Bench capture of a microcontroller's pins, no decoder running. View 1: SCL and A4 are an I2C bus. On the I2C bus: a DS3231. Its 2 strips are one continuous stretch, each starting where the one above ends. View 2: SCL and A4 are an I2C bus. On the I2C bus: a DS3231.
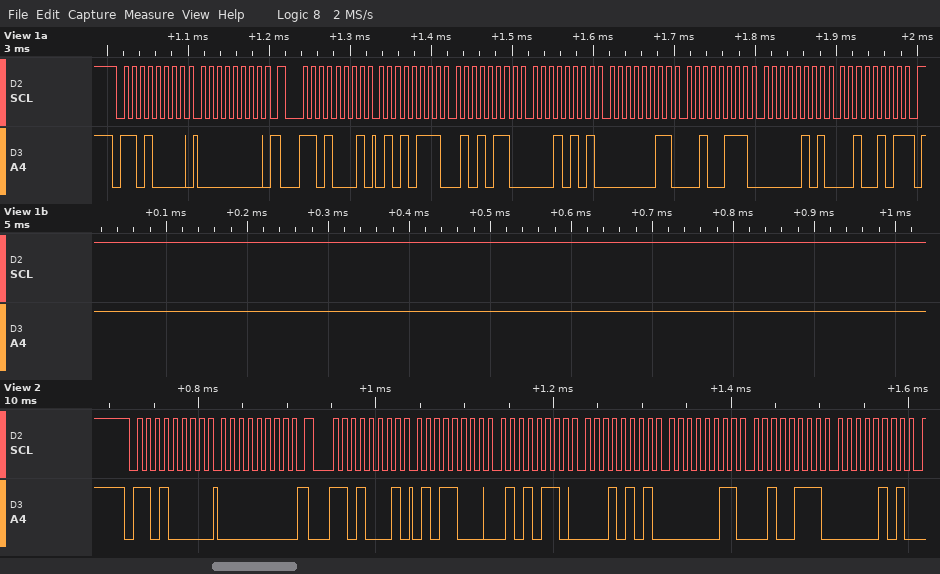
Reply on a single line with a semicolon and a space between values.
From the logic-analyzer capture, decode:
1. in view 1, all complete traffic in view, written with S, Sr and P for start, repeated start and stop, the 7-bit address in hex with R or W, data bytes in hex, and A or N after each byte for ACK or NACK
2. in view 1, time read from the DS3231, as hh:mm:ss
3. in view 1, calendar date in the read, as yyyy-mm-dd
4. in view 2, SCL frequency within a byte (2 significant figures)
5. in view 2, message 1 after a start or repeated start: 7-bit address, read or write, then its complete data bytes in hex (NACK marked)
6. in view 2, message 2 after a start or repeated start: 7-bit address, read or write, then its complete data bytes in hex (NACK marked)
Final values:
S 68W A 00 A Sr 68R A 57 A 56 A 15 A 03 A 27 A 05 A 25 N P; 15:56:57; 2025-05-27; 100 kHz; 0x68 write: 00; 0x68 read: 58 56 15 03 27 05
